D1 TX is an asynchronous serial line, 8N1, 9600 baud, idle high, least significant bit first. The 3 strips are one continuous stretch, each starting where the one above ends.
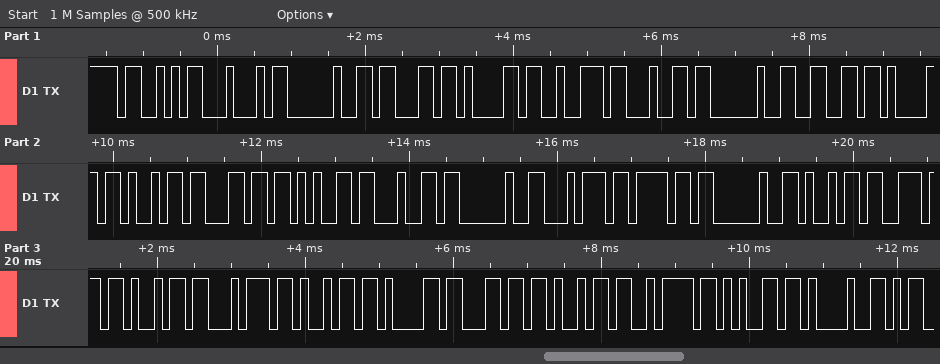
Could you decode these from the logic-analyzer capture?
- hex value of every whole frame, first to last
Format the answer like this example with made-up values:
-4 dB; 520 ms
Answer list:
0x53 0x44 0x20 0x63 0x61 0x72 0x64 0x20 0x66 0x61 0x69 0x6C 0x65 0x64 0x20 0x74 0x6F 0x20 0x69 0x6E 0x69 0x74 0x69 0x61 0x6C 0x69 0x7A 0x65 0x21
